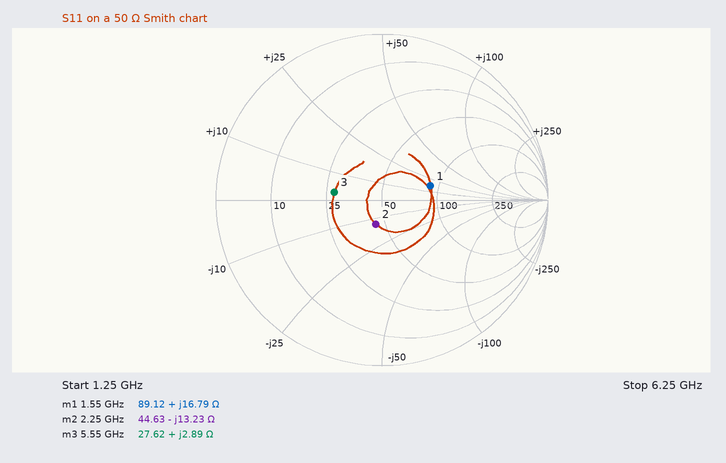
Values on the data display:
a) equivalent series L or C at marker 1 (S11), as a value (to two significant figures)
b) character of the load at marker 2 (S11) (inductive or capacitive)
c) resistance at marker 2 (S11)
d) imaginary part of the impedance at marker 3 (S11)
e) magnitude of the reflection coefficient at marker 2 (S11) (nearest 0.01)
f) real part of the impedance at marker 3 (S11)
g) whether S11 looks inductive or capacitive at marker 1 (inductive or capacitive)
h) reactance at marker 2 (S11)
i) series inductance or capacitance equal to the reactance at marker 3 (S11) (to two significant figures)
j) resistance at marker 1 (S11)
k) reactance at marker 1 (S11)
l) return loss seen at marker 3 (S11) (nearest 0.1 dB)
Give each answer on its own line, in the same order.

1.7 nH
capacitive
44.63 Ω
+2.89 Ω
0.15
27.62 Ω
inductive
-13.23 Ω
83 pH
89.12 Ω
+16.79 Ω
10.7 dB
